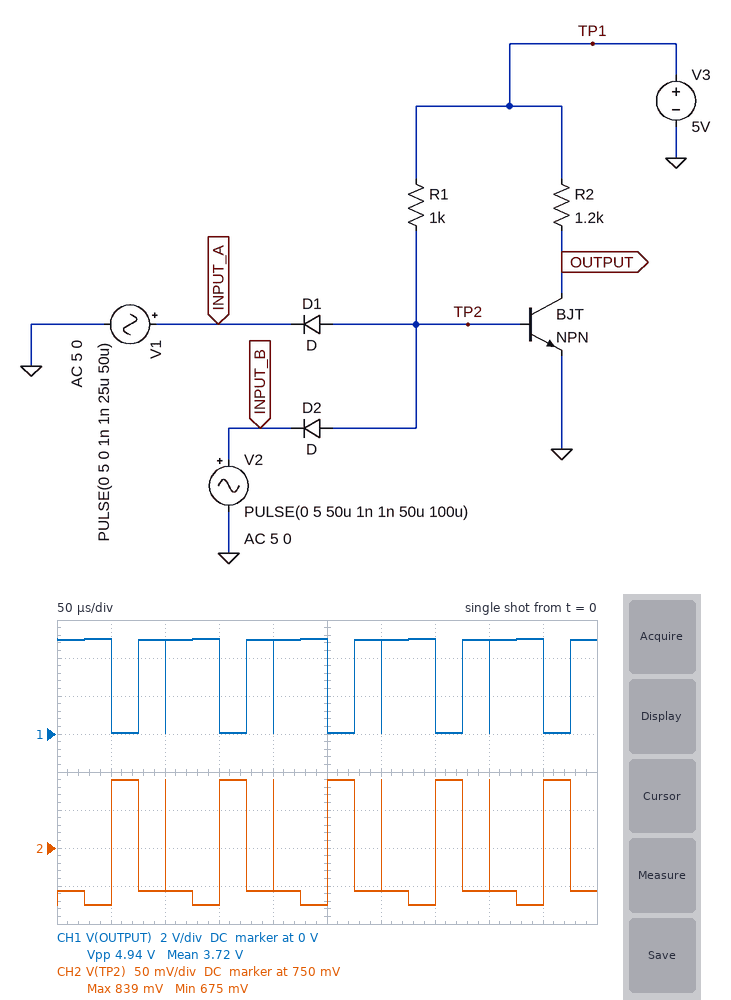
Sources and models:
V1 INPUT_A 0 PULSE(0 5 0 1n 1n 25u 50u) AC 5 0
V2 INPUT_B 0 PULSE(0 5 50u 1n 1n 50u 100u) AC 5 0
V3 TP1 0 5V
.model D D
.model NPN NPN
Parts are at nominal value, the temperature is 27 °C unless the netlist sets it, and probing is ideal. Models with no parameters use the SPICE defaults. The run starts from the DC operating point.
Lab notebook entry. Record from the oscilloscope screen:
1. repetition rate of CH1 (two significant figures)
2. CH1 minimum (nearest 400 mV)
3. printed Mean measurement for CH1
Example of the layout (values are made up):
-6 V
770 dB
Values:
10 kHz
0 V
3.72 V
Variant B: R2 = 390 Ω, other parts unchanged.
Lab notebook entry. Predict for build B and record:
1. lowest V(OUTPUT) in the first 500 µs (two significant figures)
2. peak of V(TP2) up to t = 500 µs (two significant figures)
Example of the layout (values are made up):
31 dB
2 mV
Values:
43 mV
850 mV
